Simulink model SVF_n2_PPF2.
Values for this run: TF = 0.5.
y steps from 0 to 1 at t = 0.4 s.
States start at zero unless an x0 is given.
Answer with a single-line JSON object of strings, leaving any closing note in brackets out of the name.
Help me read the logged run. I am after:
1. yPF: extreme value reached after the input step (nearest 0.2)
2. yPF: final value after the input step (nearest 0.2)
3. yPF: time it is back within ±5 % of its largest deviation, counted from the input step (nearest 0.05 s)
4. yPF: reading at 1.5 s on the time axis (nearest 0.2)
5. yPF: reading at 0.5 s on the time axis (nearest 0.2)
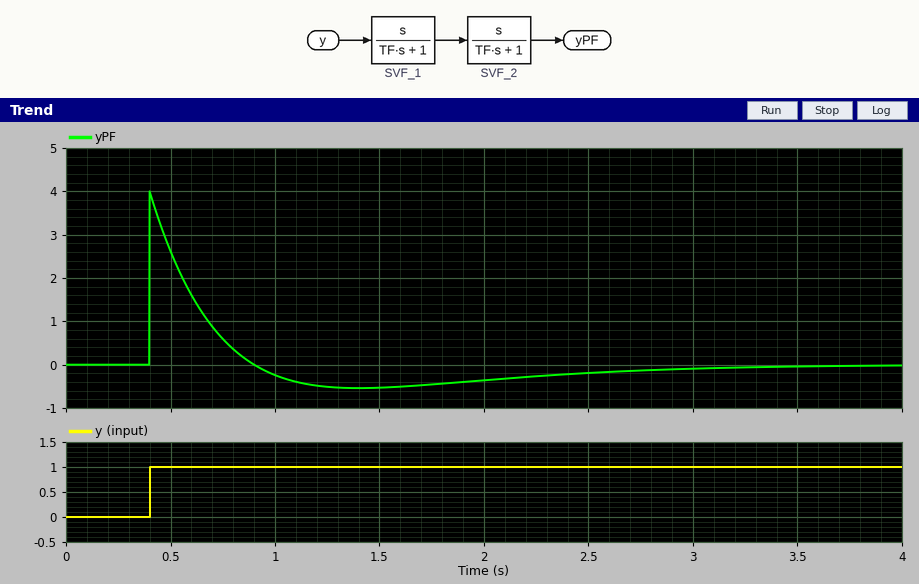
{"yPF: extreme value reached after the input step": "4.0", "yPF: final value after the input step": "0.0", "yPF: time it is back within ±5 % of its largest deviation, counted from the input step": "2.05 s", "yPF: reading at 1.5 s on the time axis": "-0.6", "yPF: reading at 0.5 s on the time axis": "2.6"}
